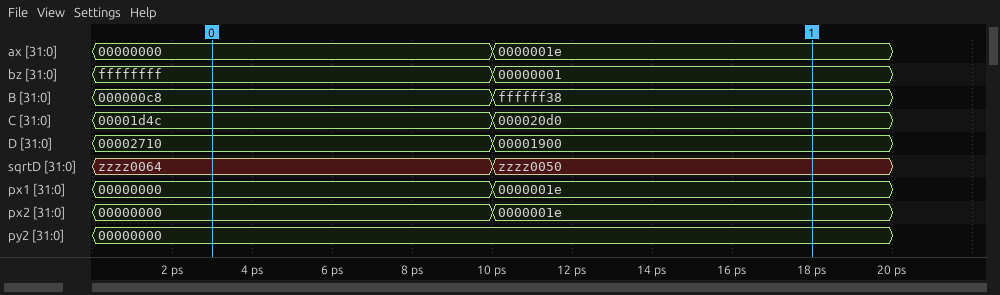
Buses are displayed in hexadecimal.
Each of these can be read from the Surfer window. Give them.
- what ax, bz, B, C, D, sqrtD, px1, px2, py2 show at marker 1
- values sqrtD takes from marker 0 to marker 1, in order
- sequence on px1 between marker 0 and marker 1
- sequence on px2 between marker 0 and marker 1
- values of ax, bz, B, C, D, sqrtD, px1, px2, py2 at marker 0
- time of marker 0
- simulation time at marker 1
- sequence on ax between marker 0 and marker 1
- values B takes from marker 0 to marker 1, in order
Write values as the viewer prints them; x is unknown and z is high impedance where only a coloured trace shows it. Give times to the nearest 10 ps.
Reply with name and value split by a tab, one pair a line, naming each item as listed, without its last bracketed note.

what ax, bz, B, C, D, sqrtD, px1, px2, py2 show at marker 1	ax=0000001e, bz=00000001, B=ffffff38, C=000020d0, D=00001900, sqrtD=zzzz0050, px1=0000001e, px2=0000001e, py2=00000000
values sqrtD takes from marker 0 to marker 1, in order	zzzz0064, zzzz0050
sequence on px1 between marker 0 and marker 1	00000000, 0000001e
sequence on px2 between marker 0 and marker 1	00000000, 0000001e
values of ax, bz, B, C, D, sqrtD, px1, px2, py2 at marker 0	ax=00000000, bz=ffffffff, B=000000c8, C=00001d4c, D=00002710, sqrtD=zzzz0064, px1=00000000, px2=00000000, py2=00000000
time of marker 0	0 ps
simulation time at marker 1	20 ps
sequence on ax between marker 0 and marker 1	00000000, 0000001e
values B takes from marker 0 to marker 1, in order	000000c8, ffffff38
